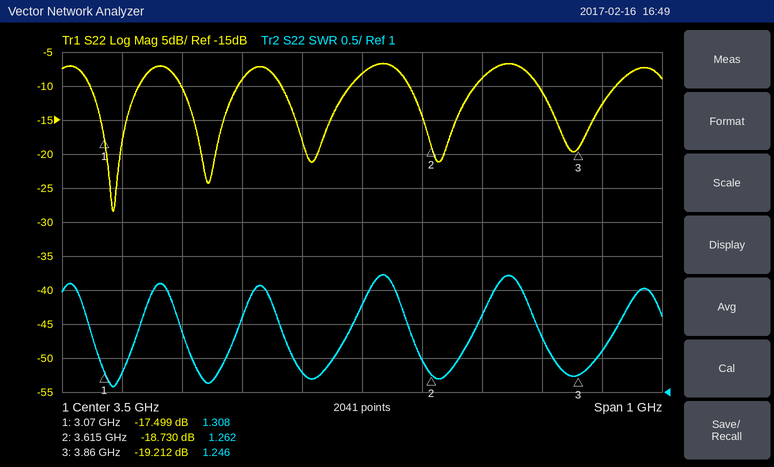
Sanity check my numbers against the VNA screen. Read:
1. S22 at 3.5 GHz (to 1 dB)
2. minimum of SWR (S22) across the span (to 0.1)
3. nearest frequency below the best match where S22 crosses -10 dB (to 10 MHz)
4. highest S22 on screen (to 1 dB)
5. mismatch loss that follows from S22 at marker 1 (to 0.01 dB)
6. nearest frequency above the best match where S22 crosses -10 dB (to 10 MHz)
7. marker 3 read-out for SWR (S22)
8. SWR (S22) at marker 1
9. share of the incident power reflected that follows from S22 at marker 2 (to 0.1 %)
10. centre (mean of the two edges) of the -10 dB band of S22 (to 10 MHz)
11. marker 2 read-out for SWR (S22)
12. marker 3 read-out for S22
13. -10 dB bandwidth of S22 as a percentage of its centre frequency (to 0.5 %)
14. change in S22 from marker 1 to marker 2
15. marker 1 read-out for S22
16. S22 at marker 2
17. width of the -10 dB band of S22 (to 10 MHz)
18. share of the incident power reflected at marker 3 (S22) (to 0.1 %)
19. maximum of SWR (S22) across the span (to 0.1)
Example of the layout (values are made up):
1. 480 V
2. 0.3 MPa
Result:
1. -8 dB
2. 1.1
3. 3.05 GHz
4. -7 dB
5. 0.08 dB
6. 3.13 GHz
7. 1.246
8. 1.308
9. 1.3 %
10. 3.09 GHz
11. 1.262
12. -19.212 dB
13. 2.5 %
14. -1.231 dB
15. -17.499 dB
16. -18.730 dB
17. 80 MHz
18. 1.2 %
19. 2.7
